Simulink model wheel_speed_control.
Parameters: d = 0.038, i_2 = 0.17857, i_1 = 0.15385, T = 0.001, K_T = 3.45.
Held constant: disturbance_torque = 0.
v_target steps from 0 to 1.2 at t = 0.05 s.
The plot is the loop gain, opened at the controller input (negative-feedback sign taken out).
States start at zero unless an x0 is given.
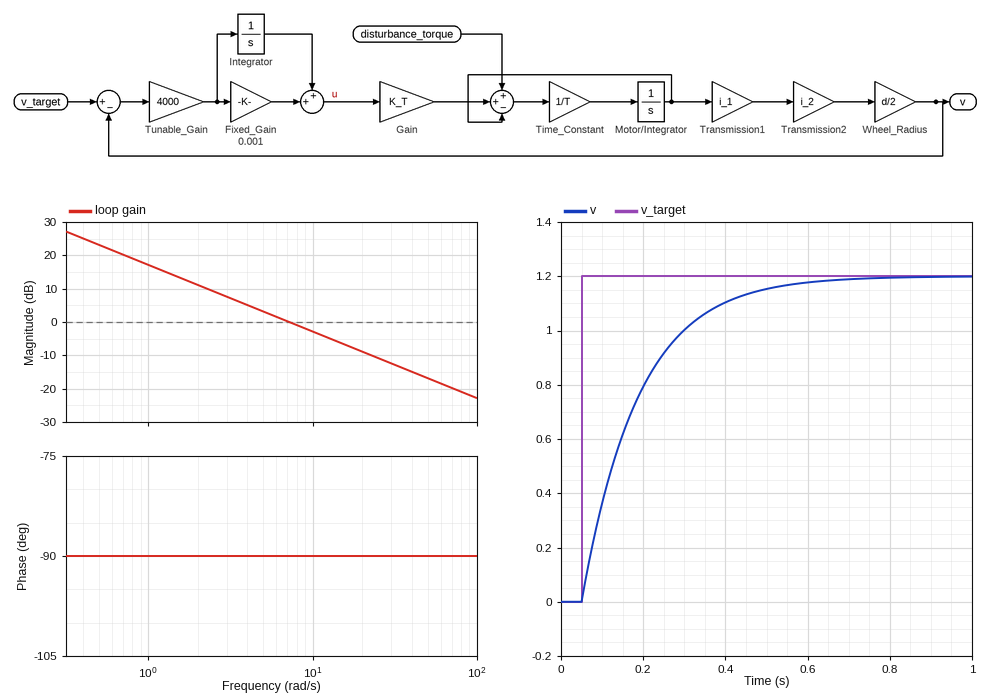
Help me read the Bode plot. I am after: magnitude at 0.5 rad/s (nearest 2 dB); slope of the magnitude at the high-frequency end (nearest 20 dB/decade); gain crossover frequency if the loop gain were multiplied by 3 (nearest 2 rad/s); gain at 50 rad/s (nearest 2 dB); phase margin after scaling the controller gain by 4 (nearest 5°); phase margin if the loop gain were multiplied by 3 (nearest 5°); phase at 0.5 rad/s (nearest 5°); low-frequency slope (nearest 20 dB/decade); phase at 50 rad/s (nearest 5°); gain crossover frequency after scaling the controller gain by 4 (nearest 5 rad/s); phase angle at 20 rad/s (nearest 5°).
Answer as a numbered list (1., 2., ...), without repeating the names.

1. 24 dB
2. -20 dB/decade
3. 22 rad/s
4. -16 dB
5. 90°
6. 90°
7. -90°
8. -20 dB/decade
9. -90°
10. 30 rad/s
11. -90°
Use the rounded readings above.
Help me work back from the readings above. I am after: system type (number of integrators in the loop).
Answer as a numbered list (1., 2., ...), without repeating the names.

1. 1
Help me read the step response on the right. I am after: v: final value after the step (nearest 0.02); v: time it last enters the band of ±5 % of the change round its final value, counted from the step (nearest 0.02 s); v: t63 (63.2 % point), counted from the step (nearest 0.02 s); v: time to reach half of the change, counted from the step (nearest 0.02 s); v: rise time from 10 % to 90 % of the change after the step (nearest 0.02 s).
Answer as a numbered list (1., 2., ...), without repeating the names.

1. 1.20
2. 0.42 s
3. 0.14 s
4. 0.10 s
5. 0.30 s
